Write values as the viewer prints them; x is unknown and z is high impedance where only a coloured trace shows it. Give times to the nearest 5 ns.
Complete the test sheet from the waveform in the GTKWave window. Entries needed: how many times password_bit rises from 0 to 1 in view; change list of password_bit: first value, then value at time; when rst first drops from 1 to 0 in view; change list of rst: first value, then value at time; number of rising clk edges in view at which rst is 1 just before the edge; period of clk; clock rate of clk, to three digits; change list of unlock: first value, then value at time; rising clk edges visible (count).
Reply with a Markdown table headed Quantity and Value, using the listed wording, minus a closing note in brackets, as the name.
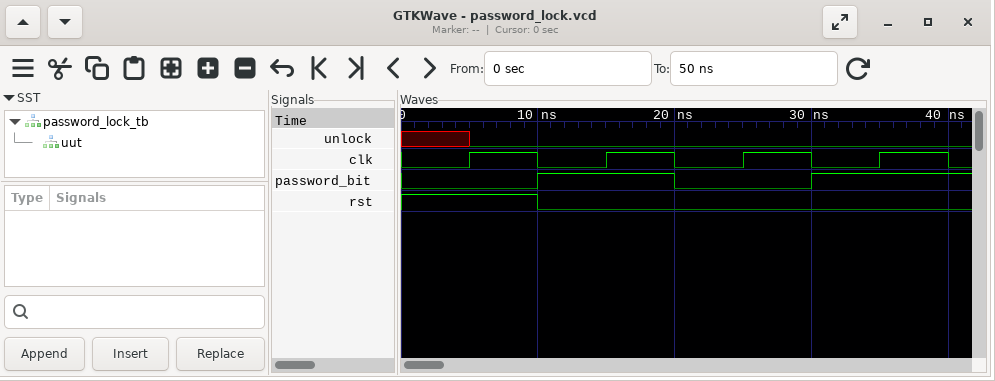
| Quantity | Value |
|---|---|
| how many times password_bit rises from 0 to 1 in view | 2 |
| change list of password_bit: first value, then value at time | 0, 1 at 10 ns, 0 at 20 ns, 1 at 30 ns |
| when rst first drops from 1 to 0 in view | 10 ns |
| change list of rst: first value, then value at time | 1, 0 at 10 ns |
| number of rising clk edges in view at which rst is 1 just before the edge | 1 |
| period of clk | 10 ns |
| clock rate of clk, to three digits | 100 MHz |
| change list of unlock: first value, then value at time | x, 0 at 5 ns |
| rising clk edges visible | 4 |
